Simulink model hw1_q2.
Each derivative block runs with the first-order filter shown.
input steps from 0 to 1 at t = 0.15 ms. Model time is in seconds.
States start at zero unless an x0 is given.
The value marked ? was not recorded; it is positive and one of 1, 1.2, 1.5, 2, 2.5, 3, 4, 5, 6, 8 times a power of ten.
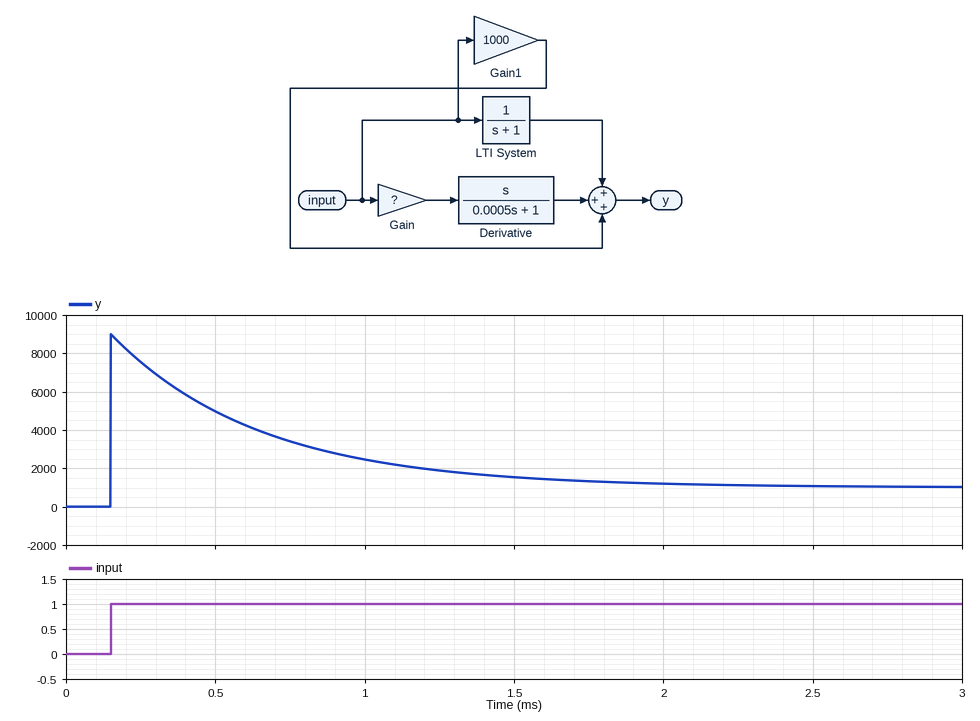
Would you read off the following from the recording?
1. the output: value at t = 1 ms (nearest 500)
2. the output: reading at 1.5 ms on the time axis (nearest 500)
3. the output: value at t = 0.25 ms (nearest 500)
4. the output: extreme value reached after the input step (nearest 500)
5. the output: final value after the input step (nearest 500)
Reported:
2500
1500
7500
9000
1000
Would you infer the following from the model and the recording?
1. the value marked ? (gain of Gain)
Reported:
4
